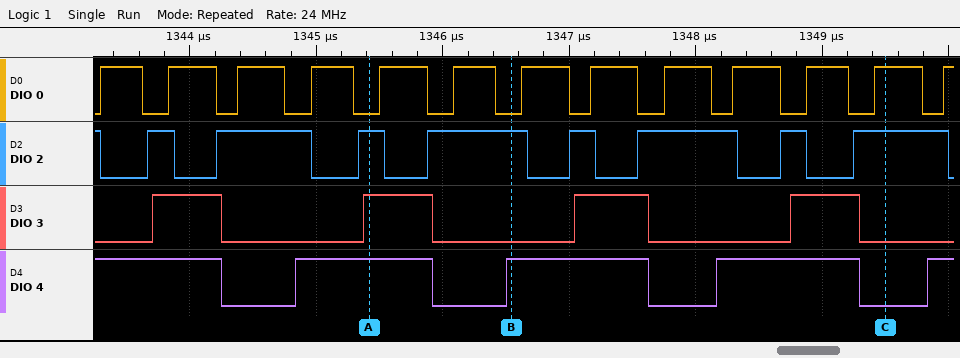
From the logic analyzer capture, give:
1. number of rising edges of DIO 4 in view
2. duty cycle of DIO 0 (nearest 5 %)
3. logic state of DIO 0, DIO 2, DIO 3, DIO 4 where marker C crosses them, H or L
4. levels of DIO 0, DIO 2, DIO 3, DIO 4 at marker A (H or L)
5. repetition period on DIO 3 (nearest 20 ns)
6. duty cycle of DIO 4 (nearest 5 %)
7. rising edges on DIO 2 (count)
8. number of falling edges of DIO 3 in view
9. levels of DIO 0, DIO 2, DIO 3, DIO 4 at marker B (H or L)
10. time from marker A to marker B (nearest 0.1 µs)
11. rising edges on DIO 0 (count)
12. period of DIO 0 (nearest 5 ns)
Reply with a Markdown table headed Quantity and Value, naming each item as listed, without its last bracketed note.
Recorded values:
| Quantity | Value |
|---|---|
| number of rising edges of DIO 4 in view | 4 |
| duty cycle of DIO 0 | 65 % |
| logic state of DIO 0, DIO 2, DIO 3, DIO 4 where marker C crosses them, H or L | DIO 0=H, DIO 2=H, DIO 3=L, DIO 4=L |
| levels of DIO 0, DIO 2, DIO 3, DIO 4 at marker A | DIO 0=L, DIO 2=H, DIO 3=H, DIO 4=H |
| repetition period on DIO 3 | 1680 ns |
| duty cycle of DIO 4 | 65 % |
| rising edges on DIO 2 | 8 |
| number of falling edges of DIO 3 in view | 4 |
| levels of DIO 0, DIO 2, DIO 3, DIO 4 at marker B | DIO 0=L, DIO 2=H, DIO 3=L, DIO 4=H |
| time from marker A to marker B | 1.1 µs |
| rising edges on DIO 0 | 13 |
| period of DIO 0 | 555 ns |
